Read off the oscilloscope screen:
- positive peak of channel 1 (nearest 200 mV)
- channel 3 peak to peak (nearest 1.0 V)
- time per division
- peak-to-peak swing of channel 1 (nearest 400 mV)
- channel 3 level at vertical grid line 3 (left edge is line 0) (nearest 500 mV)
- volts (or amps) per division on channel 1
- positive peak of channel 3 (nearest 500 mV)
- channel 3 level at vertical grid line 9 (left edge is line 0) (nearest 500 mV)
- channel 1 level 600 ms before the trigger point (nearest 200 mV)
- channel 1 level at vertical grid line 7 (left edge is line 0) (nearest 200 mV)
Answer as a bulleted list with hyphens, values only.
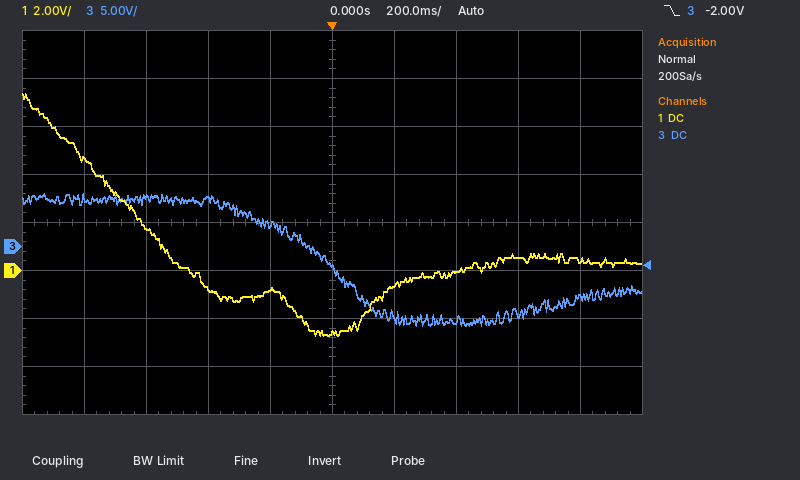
- 7.4 V
- 14.0 V
- 200 ms
- 10.0 V
- 5.0 V
- 2 V
- 5.5 V
- -5.5 V
- 1.8 V
- 0.0 V
